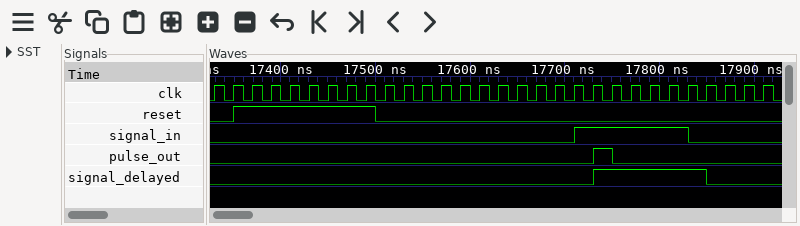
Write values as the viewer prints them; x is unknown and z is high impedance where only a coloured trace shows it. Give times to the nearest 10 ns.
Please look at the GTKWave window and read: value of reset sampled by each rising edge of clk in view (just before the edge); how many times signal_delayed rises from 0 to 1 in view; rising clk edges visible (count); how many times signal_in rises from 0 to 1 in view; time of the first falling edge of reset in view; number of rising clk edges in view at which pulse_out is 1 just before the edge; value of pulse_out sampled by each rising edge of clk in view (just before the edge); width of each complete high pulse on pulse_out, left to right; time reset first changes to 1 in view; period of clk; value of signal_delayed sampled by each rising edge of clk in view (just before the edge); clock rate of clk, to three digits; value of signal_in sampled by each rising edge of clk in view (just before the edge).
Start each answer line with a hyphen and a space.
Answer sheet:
- 0 0 1 1 1 1 1 1 1 0 0 0 0 0 0 0 0 0 0 0 0 0 0 0 0 0 0 0 0 0
- 1
- 30
- 1
- 17500 ns
- 1
- 0 0 0 0 0 0 0 0 0 0 0 0 0 0 0 0 0 0 0 0 0 1 0 0 0 0 0 0 0 0
- 20 ns
- 17350 ns
- 20 ns
- 0 0 0 0 0 0 0 0 0 0 0 0 0 0 0 0 0 0 0 0 0 1 1 1 1 1 1 0 0 0
- 50.0 MHz
- 0 0 0 0 0 0 0 0 0 0 0 0 0 0 0 0 0 0 0 0 1 1 1 1 1 1 0 0 0 0
